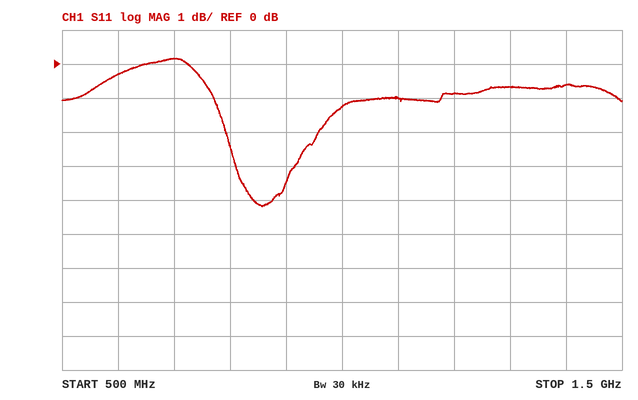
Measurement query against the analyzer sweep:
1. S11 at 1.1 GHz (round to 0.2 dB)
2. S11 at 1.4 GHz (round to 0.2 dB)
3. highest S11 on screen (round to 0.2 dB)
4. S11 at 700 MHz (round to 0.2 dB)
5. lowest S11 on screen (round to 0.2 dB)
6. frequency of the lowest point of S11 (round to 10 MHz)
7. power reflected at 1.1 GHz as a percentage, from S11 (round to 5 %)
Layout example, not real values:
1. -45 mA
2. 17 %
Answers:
1. -1.0 dB
2. -0.6 dB
3. 0.2 dB
4. 0.2 dB
5. -4.2 dB
6. 860 MHz
7. 80 %
